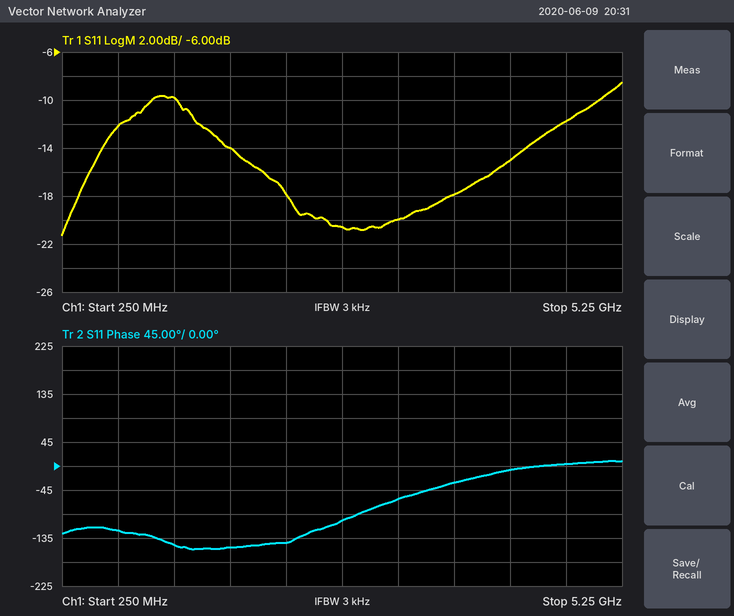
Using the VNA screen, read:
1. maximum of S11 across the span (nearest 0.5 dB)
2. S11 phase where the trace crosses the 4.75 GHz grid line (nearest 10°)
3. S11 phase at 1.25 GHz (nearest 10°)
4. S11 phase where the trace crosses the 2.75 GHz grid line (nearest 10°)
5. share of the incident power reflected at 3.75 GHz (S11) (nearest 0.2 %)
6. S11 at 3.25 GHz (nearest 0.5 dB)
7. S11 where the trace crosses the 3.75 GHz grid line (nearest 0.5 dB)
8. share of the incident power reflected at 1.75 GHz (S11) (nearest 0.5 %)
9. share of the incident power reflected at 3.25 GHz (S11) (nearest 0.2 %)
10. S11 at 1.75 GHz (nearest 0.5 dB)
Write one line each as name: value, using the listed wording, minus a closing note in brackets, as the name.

maximum of S11 across the span: -8.5 dB
S11 phase where the trace crosses the 4.75 GHz grid line: 0°
S11 phase at 1.25 GHz: -150°
S11 phase where the trace crosses the 2.75 GHz grid line: -100°
share of the incident power reflected at 3.75 GHz (S11): 1.6 %
S11 at 3.25 GHz: -20.0 dB
S11 where the trace crosses the 3.75 GHz grid line: -18.0 dB
share of the incident power reflected at 1.75 GHz (S11): 4.0 %
share of the incident power reflected at 3.25 GHz (S11): 1.0 %
S11 at 1.75 GHz: -14.0 dB
